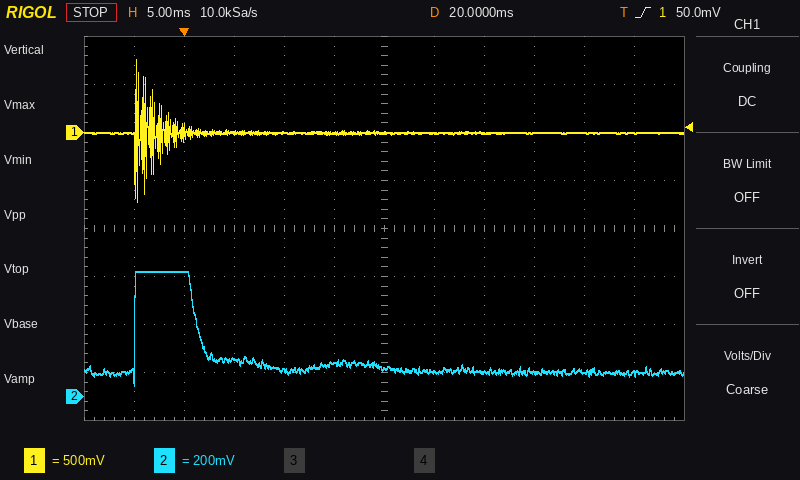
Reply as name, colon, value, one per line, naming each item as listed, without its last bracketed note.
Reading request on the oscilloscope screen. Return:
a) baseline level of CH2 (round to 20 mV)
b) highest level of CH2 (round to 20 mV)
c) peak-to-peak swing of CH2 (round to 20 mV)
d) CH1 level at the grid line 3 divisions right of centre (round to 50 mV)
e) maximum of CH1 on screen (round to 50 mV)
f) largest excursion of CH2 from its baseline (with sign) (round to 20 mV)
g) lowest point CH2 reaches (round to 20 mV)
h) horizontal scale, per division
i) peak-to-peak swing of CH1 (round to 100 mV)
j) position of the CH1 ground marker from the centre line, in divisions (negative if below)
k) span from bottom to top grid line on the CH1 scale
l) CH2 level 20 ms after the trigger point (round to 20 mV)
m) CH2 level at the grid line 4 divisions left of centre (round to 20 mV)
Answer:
baseline level of CH2: 100 mV
highest level of CH2: 520 mV
peak-to-peak swing of CH2: 480 mV
CH1 level at the grid line 3 divisions right of centre: 0 mV
maximum of CH1 on screen: 750 mV
largest excursion of CH2 from its baseline (with sign): +420 mV
lowest point CH2 reaches: 40 mV
horizontal scale, per division: 5 ms
peak-to-peak swing of CH1: 1.50 V
position of the CH1 ground marker from the centre line, in divisions: +2.0 div
span from bottom to top grid line on the CH1 scale: 4 V
CH2 level 20 ms after the trigger point: 120 mV
CH2 level at the grid line 4 divisions left of centre: 520 mV
